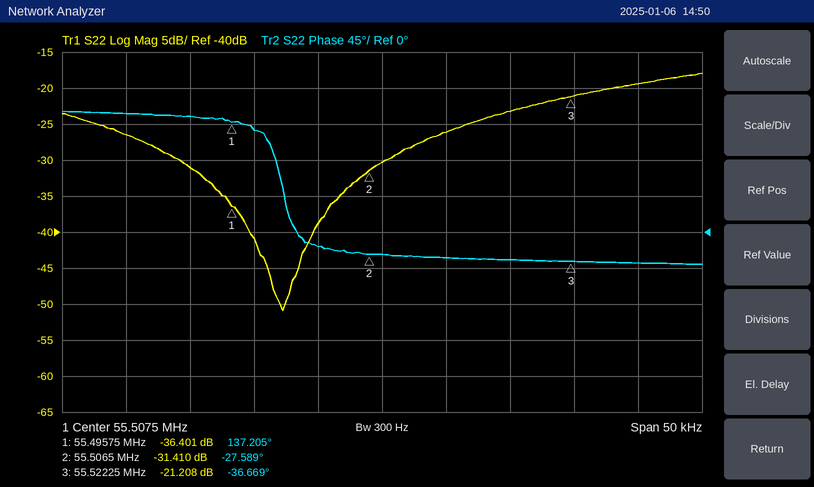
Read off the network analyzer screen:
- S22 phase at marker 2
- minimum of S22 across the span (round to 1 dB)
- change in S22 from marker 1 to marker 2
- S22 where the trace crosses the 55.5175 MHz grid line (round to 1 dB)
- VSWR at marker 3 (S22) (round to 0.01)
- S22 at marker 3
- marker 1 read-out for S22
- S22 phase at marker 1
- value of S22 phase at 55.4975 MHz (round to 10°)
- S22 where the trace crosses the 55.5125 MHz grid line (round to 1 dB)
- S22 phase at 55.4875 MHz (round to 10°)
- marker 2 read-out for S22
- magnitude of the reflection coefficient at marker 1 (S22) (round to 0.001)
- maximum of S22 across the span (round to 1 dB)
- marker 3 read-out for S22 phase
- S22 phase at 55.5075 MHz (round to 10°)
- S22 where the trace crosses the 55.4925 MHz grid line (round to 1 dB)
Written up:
-27.589°
-51 dB
4.991 dB
-23 dB
1.19
-21.208 dB
-36.401 dB
137.205°
130°
-26 dB
150°
-31.410 dB
0.015
-18 dB
-36.669°
-30°
-31 dB
